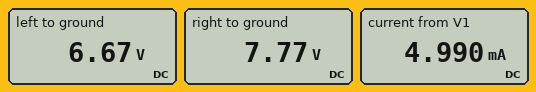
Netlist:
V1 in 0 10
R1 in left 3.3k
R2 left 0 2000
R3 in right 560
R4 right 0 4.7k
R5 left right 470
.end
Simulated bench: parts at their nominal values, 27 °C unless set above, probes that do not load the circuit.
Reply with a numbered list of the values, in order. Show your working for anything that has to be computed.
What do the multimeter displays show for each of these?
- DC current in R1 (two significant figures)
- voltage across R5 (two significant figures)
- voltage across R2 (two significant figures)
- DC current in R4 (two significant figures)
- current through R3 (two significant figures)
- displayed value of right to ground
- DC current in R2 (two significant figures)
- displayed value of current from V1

1. (10 V - 6.67 V) / 3.3 kΩ = 1.0 mA
2. 7.77 V - 6.67 V = 1.1 V
3. 6.67 V = 6.7 V
4. (7.77 V) / 4.7 kΩ = 1.7 mA
5. (10 V - 7.77 V) / 560 Ω = 4.0 mA
6. 7.77 V
7. (6.67 V) / 2 kΩ = 3.3 mA
8. 4.990 mA
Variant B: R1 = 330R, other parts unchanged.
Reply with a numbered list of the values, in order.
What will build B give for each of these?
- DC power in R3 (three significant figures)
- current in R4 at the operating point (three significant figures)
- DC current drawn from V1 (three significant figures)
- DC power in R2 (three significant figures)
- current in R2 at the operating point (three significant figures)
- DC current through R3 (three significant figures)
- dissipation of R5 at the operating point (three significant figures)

1. 2.59 mW
2. 1.87 mA
3. 6.20 mA
4. 37.5 mW
5. 4.33 mA
6. 2.15 mA
7. 37.0 µW
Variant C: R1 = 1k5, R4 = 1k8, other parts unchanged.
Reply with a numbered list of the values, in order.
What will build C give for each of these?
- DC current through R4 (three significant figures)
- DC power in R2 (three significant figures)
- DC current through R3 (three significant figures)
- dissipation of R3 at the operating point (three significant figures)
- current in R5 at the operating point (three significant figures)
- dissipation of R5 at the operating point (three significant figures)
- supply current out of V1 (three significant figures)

1. 3.98 mA
2. 22.1 mW
3. 5.07 mA
4. 14.4 mW
5. 1.09 mA
6. 559 µW
7. 7.30 mA
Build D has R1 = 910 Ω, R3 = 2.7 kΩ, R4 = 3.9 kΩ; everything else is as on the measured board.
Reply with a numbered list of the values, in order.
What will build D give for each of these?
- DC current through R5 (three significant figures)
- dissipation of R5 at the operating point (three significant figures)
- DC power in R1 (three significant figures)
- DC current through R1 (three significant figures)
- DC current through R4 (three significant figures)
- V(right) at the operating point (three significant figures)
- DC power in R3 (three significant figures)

1. 358 µA
2. 60.3 µW
3. 12.3 mW
4. 3.68 mA
5. 1.66 mA
6. 6.48 V
7. 4.59 mW
